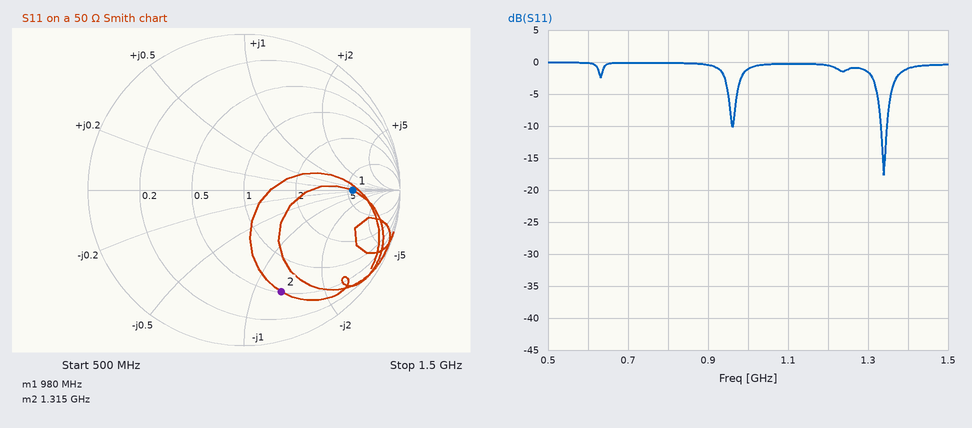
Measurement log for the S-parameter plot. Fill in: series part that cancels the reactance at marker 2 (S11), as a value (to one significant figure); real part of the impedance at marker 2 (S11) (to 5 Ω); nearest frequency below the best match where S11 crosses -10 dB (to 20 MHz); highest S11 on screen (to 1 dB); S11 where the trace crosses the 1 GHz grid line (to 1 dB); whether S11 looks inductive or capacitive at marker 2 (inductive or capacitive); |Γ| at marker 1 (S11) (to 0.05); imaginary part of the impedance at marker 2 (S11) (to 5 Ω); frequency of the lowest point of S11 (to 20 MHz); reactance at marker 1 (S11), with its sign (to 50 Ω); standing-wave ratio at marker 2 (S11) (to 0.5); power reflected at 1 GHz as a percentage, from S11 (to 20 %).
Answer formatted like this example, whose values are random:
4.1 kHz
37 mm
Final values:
8 nH
25 Ω
1.34 GHz
0 dB
-1 dB
capacitive
0.70
-65 Ω
1.34 GHz
0 Ω
5.5
80 %
